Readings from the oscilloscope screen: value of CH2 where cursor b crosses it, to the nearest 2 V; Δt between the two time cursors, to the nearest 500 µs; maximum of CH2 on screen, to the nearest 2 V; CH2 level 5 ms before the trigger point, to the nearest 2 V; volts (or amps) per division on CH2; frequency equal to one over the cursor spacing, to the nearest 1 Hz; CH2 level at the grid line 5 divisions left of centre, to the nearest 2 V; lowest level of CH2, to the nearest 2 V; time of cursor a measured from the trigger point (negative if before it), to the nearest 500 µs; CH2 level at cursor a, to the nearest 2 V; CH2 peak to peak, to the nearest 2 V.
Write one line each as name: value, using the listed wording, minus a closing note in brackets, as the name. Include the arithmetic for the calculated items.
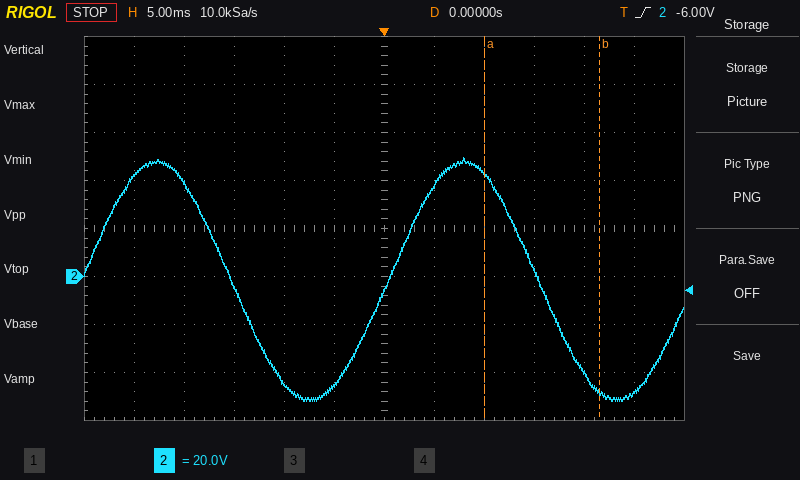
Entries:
value of CH2 where cursor b crosses it, to the nearest 2 V: -48 V
Δt between the two time cursors, to the nearest 500 µs: 11.5 ms
maximum of CH2 on screen, to the nearest 2 V: 50 V
CH2 level 5 ms before the trigger point, to the nearest 2 V: -46 V
volts (or amps) per division on CH2: 20 V
frequency equal to one over the cursor spacing, to the nearest 1 Hz: 1 / 11.5 ms ≈ 87 Hz
CH2 level at the grid line 5 divisions left of centre, to the nearest 2 V: 42 V
lowest level of CH2, to the nearest 2 V: -52 V
time of cursor a measured from the trigger point (negative if before it), to the nearest 500 µs: +10.0 ms
CH2 level at cursor a, to the nearest 2 V: 42 V
CH2 peak to peak, to the nearest 2 V: 50 V − (-52 V) = 102 V
